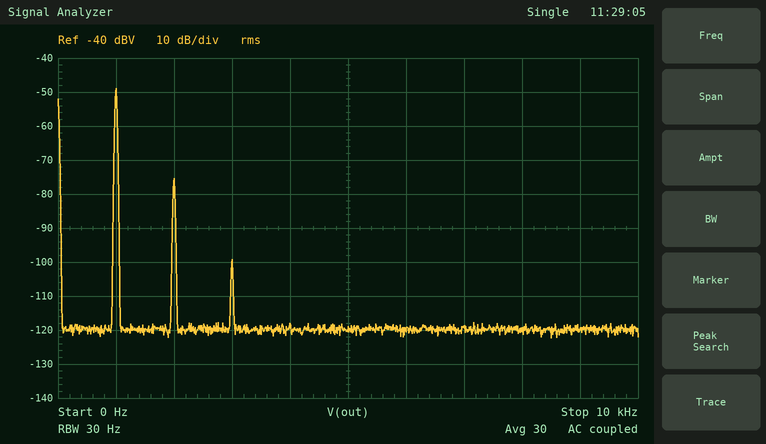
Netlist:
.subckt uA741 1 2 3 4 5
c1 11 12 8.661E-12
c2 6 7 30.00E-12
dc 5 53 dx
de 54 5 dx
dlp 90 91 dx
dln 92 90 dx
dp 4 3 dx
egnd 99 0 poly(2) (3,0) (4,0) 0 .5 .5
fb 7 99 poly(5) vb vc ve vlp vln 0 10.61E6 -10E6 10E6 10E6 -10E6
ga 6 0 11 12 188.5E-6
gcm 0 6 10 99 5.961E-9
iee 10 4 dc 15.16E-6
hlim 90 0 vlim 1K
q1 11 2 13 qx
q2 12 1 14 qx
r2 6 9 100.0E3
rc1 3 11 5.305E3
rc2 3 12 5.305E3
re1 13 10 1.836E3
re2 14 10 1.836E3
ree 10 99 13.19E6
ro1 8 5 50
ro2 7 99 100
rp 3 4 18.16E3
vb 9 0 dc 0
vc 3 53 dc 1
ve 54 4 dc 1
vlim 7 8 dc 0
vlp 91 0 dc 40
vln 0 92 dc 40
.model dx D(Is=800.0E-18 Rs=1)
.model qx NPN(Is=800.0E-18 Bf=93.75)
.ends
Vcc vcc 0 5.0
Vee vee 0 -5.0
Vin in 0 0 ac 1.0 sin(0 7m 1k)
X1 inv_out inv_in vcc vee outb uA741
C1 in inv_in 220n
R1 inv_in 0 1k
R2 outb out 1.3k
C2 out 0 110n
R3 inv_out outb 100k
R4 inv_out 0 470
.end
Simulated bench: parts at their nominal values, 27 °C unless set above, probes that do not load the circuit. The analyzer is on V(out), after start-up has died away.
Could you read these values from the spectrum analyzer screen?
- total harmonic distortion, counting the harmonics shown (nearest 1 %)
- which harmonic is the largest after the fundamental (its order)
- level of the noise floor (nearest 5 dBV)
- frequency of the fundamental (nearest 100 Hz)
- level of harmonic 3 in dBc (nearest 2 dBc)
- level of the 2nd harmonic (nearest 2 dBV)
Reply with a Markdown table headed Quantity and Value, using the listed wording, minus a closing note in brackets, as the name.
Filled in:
| Quantity | Value |
|---|---|
| total harmonic distortion, counting the harmonics shown | 5 % |
| which harmonic is the largest after the fundamental | 2 |
| level of the noise floor | -120 dBV |
| frequency of the fundamental | 1.0 kHz |
| level of harmonic 3 in dBc | -50 dBc |
| level of the 2nd harmonic | -76 dBV |
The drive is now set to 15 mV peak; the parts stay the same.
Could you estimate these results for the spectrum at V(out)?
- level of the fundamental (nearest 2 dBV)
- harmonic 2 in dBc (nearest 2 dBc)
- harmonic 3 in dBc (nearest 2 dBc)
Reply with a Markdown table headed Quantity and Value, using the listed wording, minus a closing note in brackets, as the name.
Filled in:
| Quantity | Value |
|---|---|
| level of the fundamental | -42 dBV |
| harmonic 2 in dBc | -20 dBc |
| harmonic 3 in dBc | -36 dBc |
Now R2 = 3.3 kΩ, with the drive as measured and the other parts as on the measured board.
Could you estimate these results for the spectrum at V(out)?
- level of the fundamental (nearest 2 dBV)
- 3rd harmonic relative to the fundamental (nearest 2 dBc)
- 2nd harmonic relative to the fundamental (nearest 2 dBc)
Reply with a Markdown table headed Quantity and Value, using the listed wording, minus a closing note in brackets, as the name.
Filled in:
| Quantity | Value |
|---|---|
| level of the fundamental | -54 dBV |
| 3rd harmonic relative to the fundamental | -52 dBc |
| 2nd harmonic relative to the fundamental | -28 dBc |
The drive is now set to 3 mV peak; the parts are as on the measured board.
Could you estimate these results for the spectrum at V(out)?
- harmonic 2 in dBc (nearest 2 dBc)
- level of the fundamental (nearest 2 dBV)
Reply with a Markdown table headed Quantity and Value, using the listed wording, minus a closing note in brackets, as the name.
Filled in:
| Quantity | Value |
|---|---|
| harmonic 2 in dBc | -34 dBc |
| level of the fundamental | -56 dBV |
